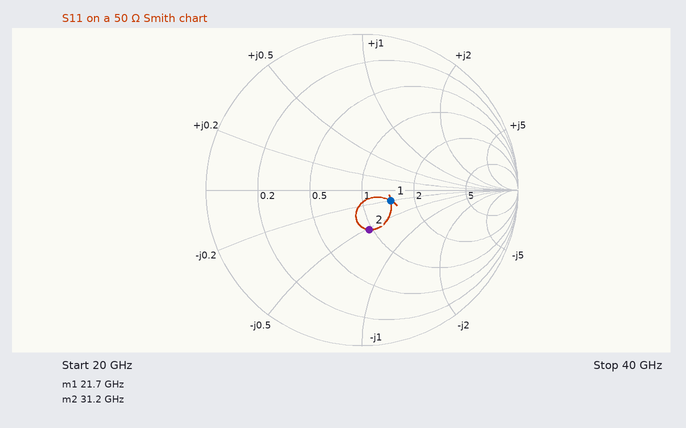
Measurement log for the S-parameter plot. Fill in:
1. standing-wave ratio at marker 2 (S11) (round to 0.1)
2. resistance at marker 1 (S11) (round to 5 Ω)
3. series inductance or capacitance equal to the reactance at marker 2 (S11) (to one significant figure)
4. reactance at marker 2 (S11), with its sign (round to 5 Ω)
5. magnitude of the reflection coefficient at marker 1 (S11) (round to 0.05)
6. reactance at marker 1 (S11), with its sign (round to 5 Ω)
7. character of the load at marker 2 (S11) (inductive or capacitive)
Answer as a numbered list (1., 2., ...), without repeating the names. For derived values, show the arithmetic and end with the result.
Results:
1. 1.7
2. 70 Ω
3. C = 1/(2π × 31.2 GHz × 25 Ω) ≈ 204 fF, so 200 fF to one significant figure
4. -25 Ω
5. 0.20
6. -10 Ω
7. capacitive
